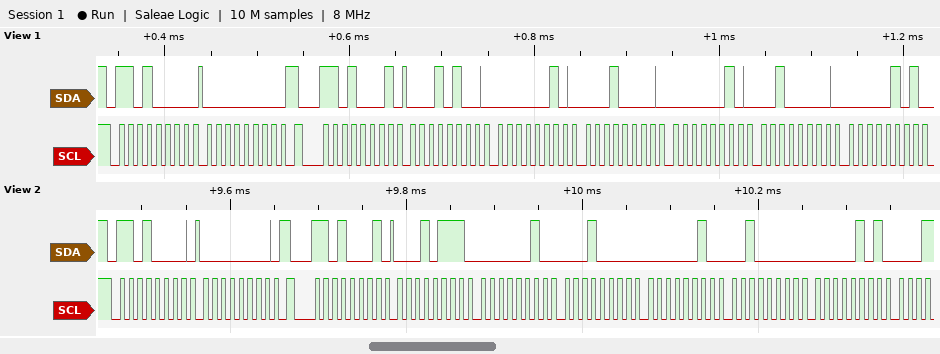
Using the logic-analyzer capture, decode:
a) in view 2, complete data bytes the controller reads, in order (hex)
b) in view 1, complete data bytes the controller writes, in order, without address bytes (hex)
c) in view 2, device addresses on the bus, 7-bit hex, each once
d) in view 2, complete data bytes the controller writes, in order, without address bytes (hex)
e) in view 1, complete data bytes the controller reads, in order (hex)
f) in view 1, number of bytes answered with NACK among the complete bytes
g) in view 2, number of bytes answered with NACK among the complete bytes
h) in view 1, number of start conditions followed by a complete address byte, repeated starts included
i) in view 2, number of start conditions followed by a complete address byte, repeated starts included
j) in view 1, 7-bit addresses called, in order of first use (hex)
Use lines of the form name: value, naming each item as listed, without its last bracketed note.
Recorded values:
in view 2, complete data bytes the controller reads, in order: 17 02 10 02 20 05
in view 1, complete data bytes the controller writes, in order, without address bytes: 00
in view 2, device addresses on the bus, 7-bit hex, each once: 0x68
in view 2, complete data bytes the controller writes, in order, without address bytes: 00
in view 1, complete data bytes the controller reads, in order: 14 02 10 02 20 05
in view 1, number of bytes answered with NACK among the complete bytes: 0
in view 2, number of bytes answered with NACK among the complete bytes: 0
in view 1, number of start conditions followed by a complete address byte, repeated starts included: 2
in view 2, number of start conditions followed by a complete address byte, repeated starts included: 2
in view 1, 7-bit addresses called, in order of first use: 0x68
